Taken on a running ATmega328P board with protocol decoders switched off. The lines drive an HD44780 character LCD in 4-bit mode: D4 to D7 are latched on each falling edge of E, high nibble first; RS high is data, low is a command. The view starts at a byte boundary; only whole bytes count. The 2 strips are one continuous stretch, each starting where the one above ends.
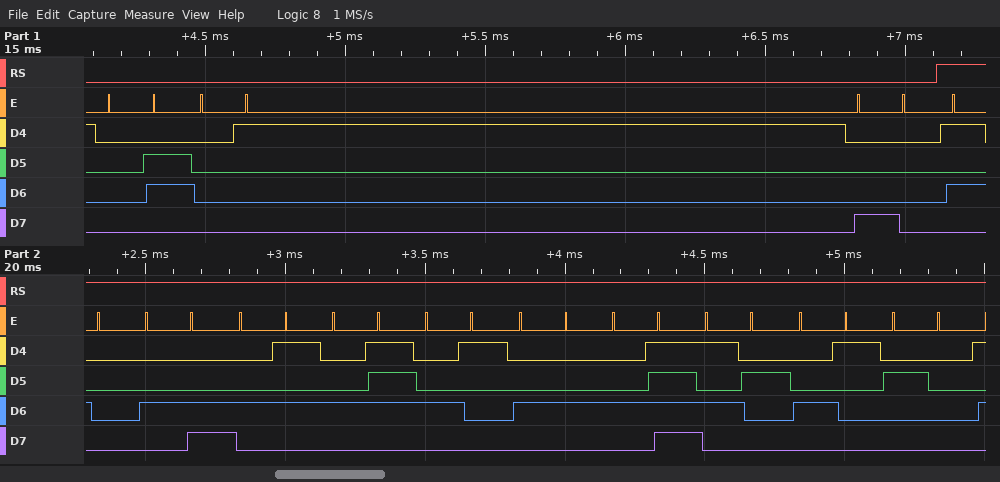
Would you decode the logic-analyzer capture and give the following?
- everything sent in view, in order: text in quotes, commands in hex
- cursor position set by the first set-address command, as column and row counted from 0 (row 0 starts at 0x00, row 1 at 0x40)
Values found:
0x06 0x01 0x80 "PLEGADORA "
column 0, row 0
